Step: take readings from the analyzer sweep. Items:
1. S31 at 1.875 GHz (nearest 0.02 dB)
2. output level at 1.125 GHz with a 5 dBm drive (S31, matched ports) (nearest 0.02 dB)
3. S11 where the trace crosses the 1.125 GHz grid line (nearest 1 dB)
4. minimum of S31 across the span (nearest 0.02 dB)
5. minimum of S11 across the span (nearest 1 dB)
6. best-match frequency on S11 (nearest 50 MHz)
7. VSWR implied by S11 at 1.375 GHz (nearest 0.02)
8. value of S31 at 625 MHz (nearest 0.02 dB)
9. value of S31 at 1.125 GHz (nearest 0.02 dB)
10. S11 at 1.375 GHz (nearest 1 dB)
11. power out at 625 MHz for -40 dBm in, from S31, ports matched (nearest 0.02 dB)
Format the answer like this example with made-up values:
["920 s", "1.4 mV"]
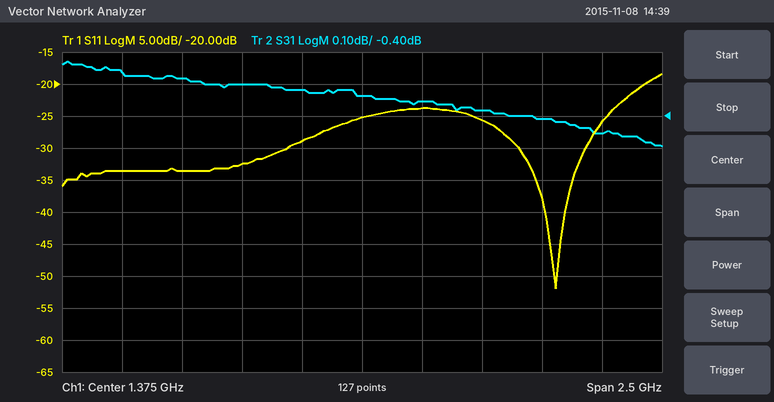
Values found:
["-0.38 dB", "4.68 dBm", "-29 dB", "-0.50 dB", "-52 dB", "2.20 GHz", "1.12", "-0.28 dB", "-0.32 dB", "-25 dB", "-40.28 dBm"]
